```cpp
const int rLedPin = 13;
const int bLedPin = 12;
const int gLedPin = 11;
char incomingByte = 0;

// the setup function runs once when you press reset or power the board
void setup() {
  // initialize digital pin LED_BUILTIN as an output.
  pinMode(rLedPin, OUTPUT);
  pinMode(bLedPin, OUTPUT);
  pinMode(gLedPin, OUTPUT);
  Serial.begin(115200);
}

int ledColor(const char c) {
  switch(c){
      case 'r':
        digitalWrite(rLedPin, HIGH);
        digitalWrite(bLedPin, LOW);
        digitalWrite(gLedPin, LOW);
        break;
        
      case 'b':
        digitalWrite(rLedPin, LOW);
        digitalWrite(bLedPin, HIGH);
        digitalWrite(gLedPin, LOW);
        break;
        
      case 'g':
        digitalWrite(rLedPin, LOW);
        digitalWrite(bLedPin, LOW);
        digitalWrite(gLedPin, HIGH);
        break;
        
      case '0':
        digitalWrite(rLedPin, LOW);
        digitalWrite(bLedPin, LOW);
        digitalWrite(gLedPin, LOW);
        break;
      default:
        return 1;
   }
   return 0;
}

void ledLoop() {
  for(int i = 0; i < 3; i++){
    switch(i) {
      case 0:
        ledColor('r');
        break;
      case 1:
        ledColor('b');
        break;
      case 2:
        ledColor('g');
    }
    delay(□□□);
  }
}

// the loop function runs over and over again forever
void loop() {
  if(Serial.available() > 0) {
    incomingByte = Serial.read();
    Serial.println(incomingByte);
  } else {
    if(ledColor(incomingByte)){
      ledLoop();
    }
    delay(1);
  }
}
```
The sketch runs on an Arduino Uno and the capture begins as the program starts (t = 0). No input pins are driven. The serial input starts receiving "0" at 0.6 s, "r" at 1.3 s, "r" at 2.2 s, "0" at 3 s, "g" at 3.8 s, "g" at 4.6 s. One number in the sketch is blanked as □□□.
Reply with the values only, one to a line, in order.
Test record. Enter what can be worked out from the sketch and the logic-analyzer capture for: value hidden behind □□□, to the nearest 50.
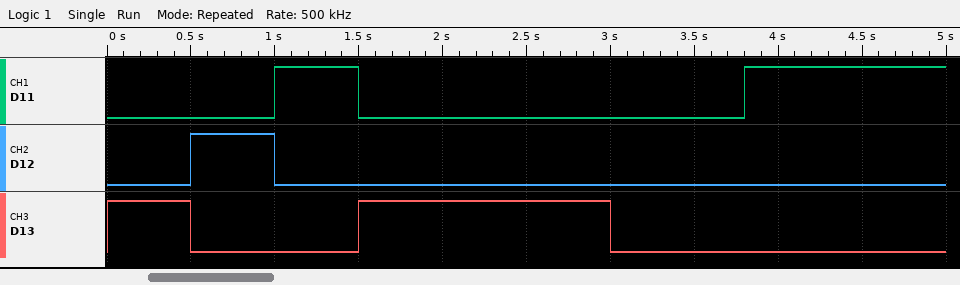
500
